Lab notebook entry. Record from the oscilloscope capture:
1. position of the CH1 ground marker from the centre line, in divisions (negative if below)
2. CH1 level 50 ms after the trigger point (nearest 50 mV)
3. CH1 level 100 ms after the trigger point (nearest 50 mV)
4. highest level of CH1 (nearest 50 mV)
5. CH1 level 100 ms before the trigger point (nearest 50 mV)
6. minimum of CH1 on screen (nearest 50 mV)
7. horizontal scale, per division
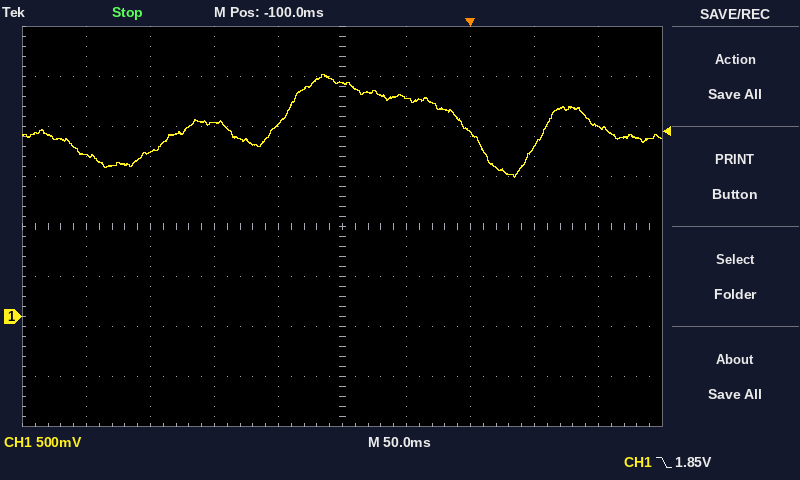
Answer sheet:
-1.8 div
1.70 V
1.90 V
2.40 V
2.35 V
1.40 V
50 ms
